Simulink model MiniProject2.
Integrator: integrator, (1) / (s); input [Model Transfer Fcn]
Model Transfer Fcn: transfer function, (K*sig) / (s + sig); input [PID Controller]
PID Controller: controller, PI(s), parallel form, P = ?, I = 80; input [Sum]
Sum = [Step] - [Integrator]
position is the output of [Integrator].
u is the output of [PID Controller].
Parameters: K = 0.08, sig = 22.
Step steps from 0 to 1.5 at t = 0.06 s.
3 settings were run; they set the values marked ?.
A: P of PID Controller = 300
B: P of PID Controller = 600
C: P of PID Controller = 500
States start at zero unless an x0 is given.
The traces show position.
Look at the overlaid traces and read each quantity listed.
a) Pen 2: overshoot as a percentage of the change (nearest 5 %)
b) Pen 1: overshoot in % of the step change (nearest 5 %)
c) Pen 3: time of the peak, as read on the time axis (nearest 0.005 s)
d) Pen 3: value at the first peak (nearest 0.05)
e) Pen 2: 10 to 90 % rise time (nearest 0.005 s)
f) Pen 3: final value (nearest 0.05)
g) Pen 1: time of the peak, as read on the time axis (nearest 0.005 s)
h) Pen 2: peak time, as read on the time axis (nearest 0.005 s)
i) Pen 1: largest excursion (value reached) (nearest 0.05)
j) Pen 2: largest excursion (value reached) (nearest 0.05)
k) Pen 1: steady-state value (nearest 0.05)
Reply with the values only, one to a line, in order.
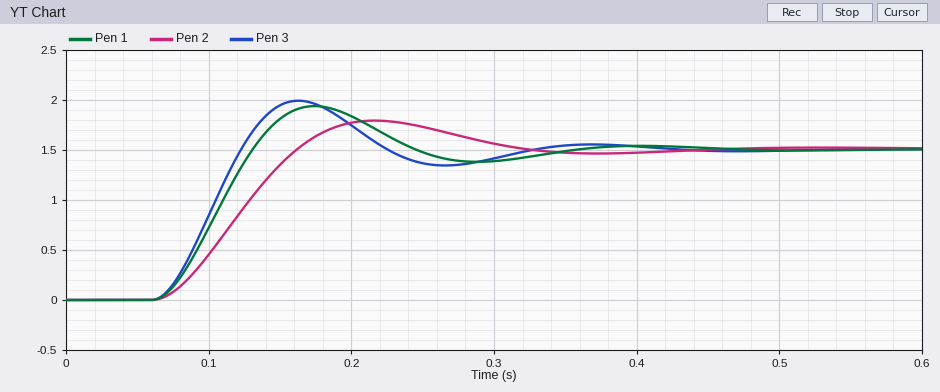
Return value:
20 %
30 %
0.165 s
2.00
0.070 s
1.50
0.175 s
0.215 s
1.95
1.80
1.50
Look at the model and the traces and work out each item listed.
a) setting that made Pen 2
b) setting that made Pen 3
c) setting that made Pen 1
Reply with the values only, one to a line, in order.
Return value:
A
B
C
